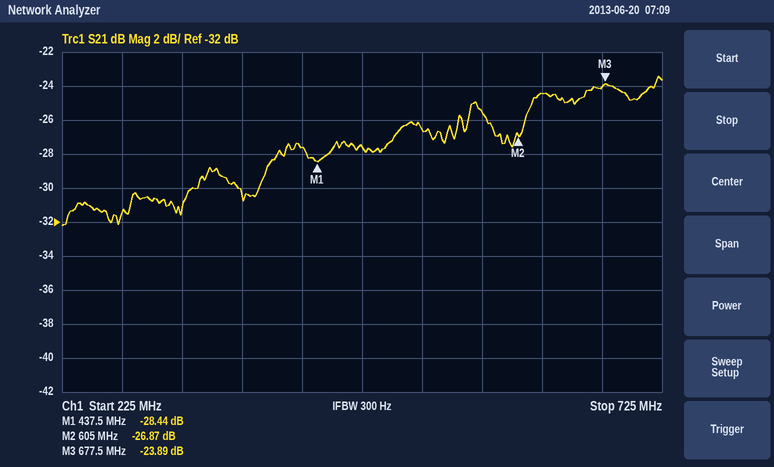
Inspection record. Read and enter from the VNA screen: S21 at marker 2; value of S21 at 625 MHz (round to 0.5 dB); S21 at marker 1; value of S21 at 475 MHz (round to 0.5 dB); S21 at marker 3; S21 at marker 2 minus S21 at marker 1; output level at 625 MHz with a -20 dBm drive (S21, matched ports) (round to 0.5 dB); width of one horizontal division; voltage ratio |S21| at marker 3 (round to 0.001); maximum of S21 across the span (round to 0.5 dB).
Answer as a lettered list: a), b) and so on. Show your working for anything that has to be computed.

a) -26.87 dB
b) -24.5 dB
c) -28.44 dB
d) -27.5 dB
e) -23.89 dB
f) -26.87 − (-28.44) = 1.57 dB
g) -20 dBm + (-24.5 dB) = -44.5 dBm
h) 50 MHz
i) 10^(-23.89/20) ≈ 0.064
j) -23.5 dB
